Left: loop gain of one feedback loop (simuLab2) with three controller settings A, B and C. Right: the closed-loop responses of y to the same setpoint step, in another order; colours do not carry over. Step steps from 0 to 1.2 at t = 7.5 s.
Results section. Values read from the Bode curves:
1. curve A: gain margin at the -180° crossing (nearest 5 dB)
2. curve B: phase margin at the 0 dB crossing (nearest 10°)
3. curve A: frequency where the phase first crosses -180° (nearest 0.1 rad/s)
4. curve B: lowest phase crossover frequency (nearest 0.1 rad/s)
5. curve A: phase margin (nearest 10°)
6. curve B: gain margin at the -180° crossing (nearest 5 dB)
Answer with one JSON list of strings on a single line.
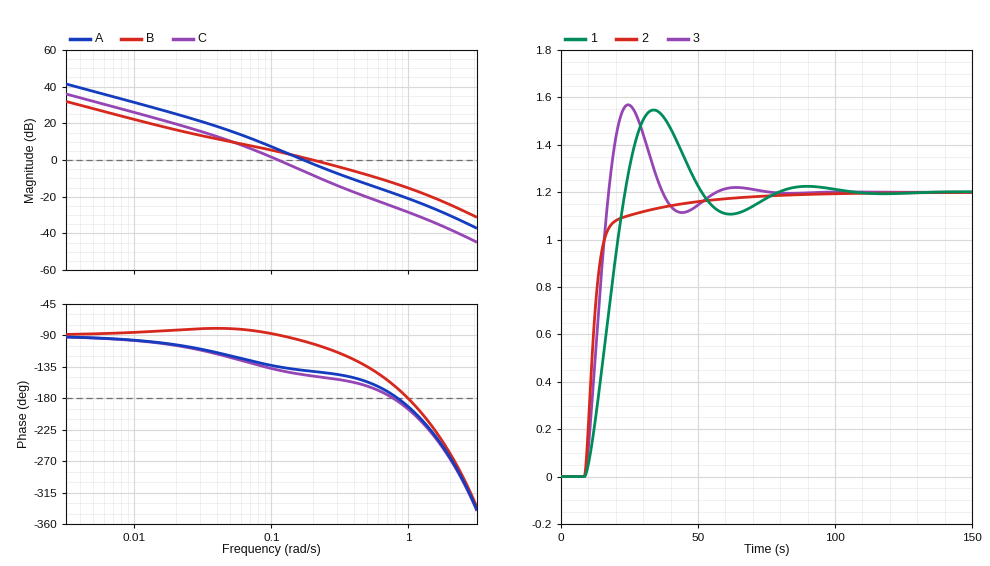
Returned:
["20 dB", "80°", "0.8 rad/s", "1.0 rad/s", "40°", "15 dB"]
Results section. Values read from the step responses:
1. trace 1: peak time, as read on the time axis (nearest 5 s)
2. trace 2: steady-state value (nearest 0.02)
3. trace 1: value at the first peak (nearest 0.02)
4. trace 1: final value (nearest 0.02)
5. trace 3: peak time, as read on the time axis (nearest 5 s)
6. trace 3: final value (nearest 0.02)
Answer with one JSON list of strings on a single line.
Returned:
["35 s", "1.20", "1.54", "1.20", "25 s", "1.20"]
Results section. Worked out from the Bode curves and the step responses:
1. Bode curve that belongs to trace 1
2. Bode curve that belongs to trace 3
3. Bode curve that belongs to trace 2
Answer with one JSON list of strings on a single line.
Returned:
["C", "A", "B"]
